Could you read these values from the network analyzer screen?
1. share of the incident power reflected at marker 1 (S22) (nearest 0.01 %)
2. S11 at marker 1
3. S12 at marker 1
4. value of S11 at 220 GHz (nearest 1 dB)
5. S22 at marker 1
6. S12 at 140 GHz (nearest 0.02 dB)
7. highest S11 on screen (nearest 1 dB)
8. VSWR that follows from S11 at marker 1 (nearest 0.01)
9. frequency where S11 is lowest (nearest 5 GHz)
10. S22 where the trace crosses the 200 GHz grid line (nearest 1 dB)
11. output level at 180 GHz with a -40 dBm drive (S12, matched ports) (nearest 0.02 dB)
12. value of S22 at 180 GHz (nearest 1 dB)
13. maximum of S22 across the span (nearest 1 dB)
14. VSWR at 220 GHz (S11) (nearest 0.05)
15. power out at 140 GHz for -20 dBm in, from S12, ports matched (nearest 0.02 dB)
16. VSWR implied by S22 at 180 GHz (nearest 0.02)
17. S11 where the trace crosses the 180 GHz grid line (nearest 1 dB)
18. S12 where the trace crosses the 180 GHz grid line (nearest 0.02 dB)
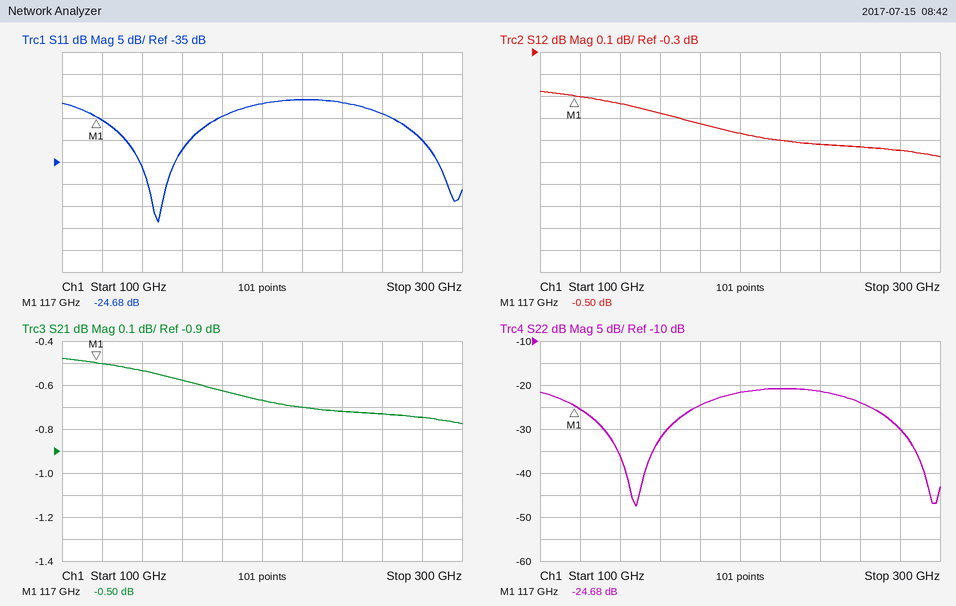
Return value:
0.34 %
-24.68 dB
-0.50 dB
-21 dB
-24.68 dB
-0.54 dB
-21 dB
1.12
150 GHz
-22 dB
-40.62 dBm
-25 dB
-21 dB
1.20
-20.54 dBm
1.12
-25 dB
-0.62 dB
